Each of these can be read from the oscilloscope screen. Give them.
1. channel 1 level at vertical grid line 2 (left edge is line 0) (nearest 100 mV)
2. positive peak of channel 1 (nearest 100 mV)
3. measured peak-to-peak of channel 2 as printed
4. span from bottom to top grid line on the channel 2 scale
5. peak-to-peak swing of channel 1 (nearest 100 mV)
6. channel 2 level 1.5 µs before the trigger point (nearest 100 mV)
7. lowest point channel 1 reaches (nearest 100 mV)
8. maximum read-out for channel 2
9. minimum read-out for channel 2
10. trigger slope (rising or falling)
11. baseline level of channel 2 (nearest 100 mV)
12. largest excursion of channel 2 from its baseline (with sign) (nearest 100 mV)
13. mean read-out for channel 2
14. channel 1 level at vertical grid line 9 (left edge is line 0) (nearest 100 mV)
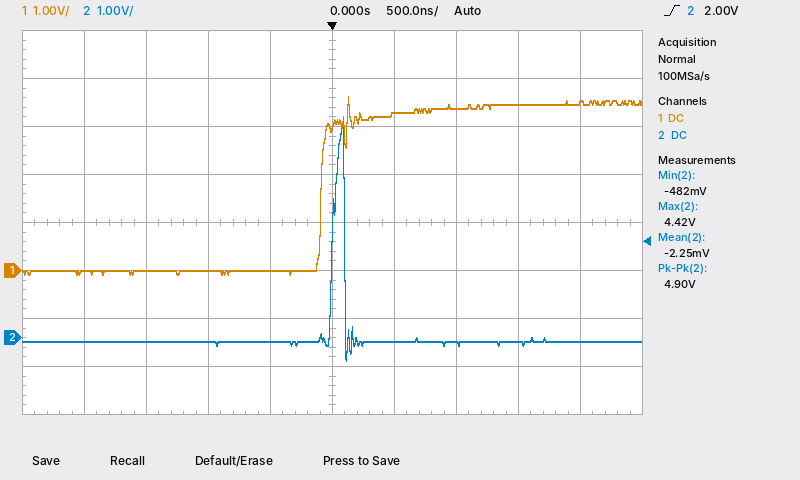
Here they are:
0.0 V
3.6 V
4.90 V
8 V
3.7 V
-100 mV
-100 mV
4.42 V
-482 mV
rising
-100 mV
+4.5 V
-2.25 mV
3.5 V
